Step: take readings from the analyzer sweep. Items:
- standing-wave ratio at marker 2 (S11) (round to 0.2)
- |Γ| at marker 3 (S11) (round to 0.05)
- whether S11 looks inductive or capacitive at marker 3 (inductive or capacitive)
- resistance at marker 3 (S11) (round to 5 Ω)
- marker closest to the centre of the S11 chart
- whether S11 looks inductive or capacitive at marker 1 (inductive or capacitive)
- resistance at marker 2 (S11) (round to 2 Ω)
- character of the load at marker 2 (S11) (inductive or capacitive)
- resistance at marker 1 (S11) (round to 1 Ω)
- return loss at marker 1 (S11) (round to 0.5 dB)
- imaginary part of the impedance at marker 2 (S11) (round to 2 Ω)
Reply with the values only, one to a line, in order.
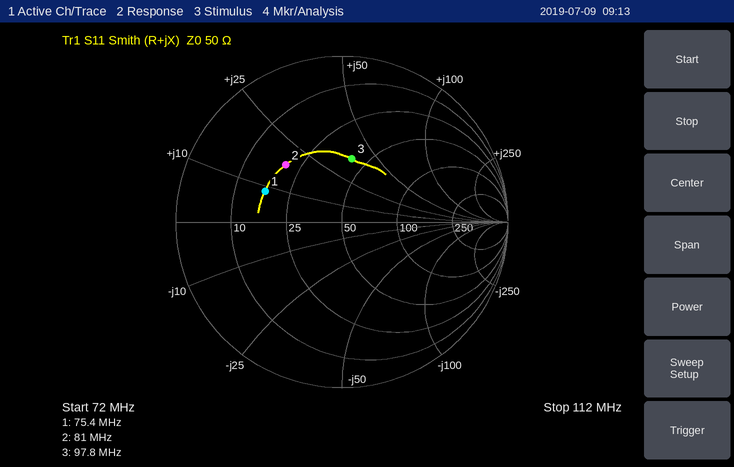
2.8
0.40
inductive
40 Ω
marker 3
inductive
20 Ω
inductive
17 Ω
6.0 dB
+18 Ω
